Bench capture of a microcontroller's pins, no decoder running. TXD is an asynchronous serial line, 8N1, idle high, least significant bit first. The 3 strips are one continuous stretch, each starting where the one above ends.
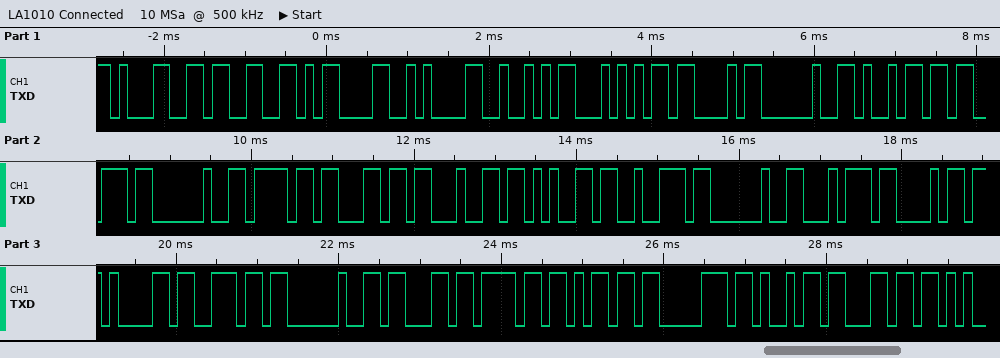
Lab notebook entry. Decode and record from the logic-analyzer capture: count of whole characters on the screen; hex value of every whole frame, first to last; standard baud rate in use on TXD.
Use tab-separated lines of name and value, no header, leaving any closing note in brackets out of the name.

count of whole characters on the screen	28
hex value of every whole frame, first to last	31 33 0D 0A 52 54 43 20 69 73 20 6F 6C 64 65 72 20 74 68 61 6E 20 63 6F 6D 70 69 6C
standard baud rate in use on TXD	9600 baud
